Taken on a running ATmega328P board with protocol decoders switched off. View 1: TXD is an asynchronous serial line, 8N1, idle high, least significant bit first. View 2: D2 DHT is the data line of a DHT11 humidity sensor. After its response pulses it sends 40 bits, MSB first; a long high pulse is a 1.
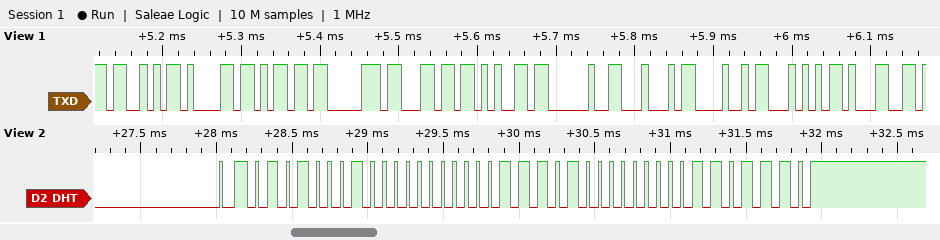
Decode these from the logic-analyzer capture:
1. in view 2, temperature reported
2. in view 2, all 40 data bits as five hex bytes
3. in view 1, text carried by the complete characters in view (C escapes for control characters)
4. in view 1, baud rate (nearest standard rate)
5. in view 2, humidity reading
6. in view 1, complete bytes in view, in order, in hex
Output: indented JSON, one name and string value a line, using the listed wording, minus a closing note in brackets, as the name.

{
  "in view 2, temperature reported": "29.0 °C",
  "in view 2, all 40 data bits as five hex bytes": "51 00 1D 00 6E",
  "in view 1, text carried by the complete characters in view": "\"Sample DHT1\"",
  "in view 1, baud rate": "115200 baud",
  "in view 2, humidity reading": "81 %",
  "in view 1, complete bytes in view, in order, in hex": "0x53 0x61 0x6D 0x70 0x6C 0x65 0x20 0x44 0x48 0x54 0x31"
}
